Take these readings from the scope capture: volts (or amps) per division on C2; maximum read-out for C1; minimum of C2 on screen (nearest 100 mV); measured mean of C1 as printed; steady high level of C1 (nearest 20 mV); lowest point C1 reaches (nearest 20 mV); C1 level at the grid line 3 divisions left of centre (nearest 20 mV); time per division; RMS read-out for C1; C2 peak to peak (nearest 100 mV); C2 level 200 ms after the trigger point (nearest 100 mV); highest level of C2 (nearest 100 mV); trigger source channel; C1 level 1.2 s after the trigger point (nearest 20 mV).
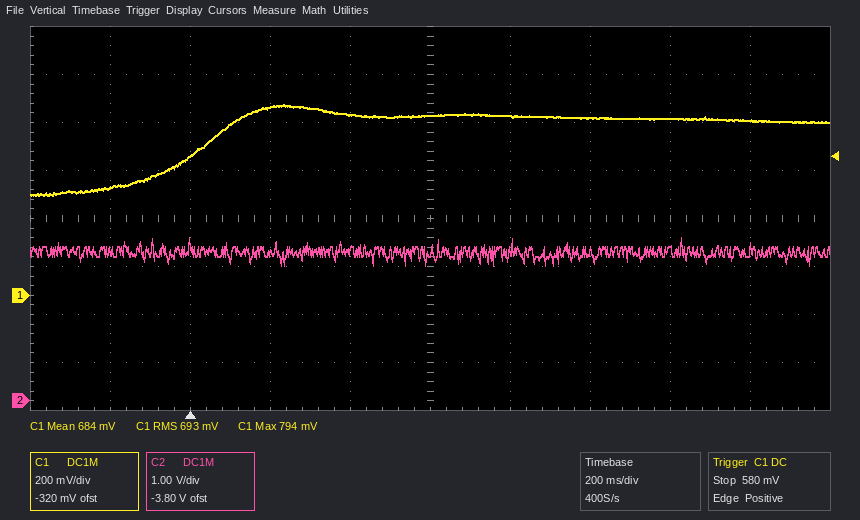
1 V
794 mV
2.8 V
684 mV
740 mV
420 mV
580 mV
200 ms
693 mV
600 mV
3.1 V
3.4 V
C1
740 mV
